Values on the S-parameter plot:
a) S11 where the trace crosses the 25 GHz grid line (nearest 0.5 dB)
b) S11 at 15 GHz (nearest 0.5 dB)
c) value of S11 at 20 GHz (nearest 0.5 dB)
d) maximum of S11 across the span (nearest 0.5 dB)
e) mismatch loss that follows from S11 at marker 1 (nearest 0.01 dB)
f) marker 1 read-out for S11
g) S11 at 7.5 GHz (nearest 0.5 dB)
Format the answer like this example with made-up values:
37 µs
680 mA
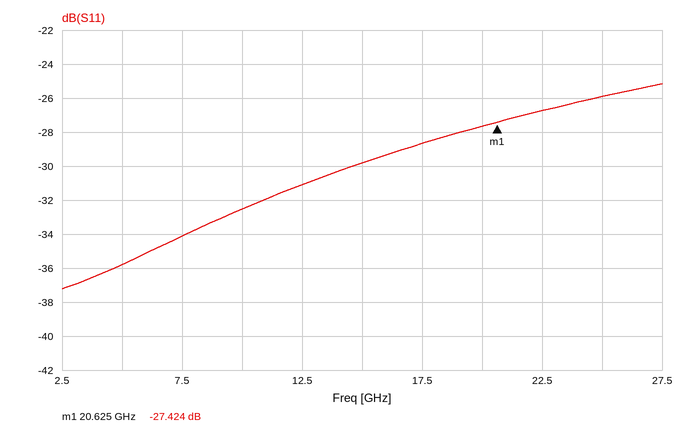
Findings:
-26.0 dB
-30.0 dB
-27.5 dB
-25.0 dB
0.01 dB
-27.424 dB
-34.0 dB
